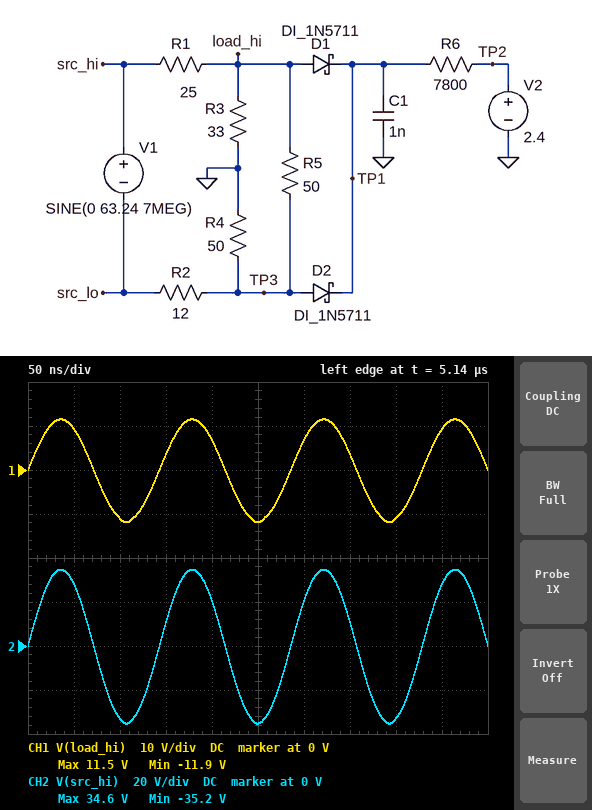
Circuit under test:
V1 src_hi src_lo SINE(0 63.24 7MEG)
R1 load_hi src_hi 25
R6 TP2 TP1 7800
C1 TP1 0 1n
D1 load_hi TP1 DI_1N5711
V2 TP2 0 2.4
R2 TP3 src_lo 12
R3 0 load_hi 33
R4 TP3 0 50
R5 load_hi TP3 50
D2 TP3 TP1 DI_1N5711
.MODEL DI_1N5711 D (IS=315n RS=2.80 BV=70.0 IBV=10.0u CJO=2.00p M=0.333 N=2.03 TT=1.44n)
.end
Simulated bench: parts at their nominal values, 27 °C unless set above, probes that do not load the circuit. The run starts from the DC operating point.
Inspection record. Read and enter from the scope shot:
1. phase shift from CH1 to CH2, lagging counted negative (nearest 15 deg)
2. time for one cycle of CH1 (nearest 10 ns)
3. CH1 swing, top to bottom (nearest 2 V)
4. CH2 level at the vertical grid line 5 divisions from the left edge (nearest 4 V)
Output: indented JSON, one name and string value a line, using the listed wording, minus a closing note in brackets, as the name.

{
  "phase shift from CH1 to CH2, lagging counted negative": "0 deg",
  "time for one cycle of CH1": "140 ns",
  "CH1 swing, top to bottom": "24 V",
  "CH2 level at the vertical grid line 5 divisions from the left edge": "-36 V"
}
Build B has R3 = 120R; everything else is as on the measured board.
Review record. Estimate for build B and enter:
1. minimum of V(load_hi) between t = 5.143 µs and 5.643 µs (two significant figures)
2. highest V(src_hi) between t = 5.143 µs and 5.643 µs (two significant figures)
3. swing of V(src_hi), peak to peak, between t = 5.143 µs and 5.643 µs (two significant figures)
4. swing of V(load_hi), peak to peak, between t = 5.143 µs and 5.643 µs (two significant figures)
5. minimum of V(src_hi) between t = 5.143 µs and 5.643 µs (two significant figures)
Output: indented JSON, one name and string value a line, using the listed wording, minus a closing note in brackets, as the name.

{
  "minimum of V(load_hi) between t = 5.143 µs and 5.643 µs": "-23 V",
  "highest V(src_hi) between t = 5.143 µs and 5.643 µs": "43 V",
  "swing of V(src_hi), peak to peak, between t = 5.143 µs and 5.643 µs": "86 V",
  "swing of V(load_hi), peak to peak, between t = 5.143 µs and 5.643 µs": "44 V",
  "minimum of V(src_hi) between t = 5.143 µs and 5.643 µs": "-44 V"
}
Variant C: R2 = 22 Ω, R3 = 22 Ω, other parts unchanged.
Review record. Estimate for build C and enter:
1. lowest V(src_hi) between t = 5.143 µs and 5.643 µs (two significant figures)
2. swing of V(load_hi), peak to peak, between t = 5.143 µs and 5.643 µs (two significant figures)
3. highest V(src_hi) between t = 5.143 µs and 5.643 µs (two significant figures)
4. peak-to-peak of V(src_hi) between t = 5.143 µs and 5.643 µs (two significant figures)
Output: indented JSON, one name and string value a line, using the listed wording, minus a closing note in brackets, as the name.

{
  "lowest V(src_hi) between t = 5.143 µs and 5.643 µs": "-29 V",
  "swing of V(load_hi), peak to peak, between t = 5.143 µs and 5.643 µs": "15 V",
  "highest V(src_hi) between t = 5.143 µs and 5.643 µs": "28 V",
  "peak-to-peak of V(src_hi) between t = 5.143 µs and 5.643 µs": "57 V"
}
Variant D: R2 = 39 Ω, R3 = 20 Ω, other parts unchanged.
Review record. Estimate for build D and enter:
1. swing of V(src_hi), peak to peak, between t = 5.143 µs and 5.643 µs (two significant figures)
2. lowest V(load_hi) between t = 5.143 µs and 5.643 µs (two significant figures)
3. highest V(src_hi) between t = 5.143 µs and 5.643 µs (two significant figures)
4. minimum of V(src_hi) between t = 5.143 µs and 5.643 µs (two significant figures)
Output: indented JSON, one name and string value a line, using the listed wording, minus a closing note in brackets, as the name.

{
  "swing of V(src_hi), peak to peak, between t = 5.143 µs and 5.643 µs": "46 V",
  "lowest V(load_hi) between t = 5.143 µs and 5.643 µs": "-5.9 V",
  "highest V(src_hi) between t = 5.143 µs and 5.643 µs": "23 V",
  "minimum of V(src_hi) between t = 5.143 µs and 5.643 µs": "-23 V"
}
